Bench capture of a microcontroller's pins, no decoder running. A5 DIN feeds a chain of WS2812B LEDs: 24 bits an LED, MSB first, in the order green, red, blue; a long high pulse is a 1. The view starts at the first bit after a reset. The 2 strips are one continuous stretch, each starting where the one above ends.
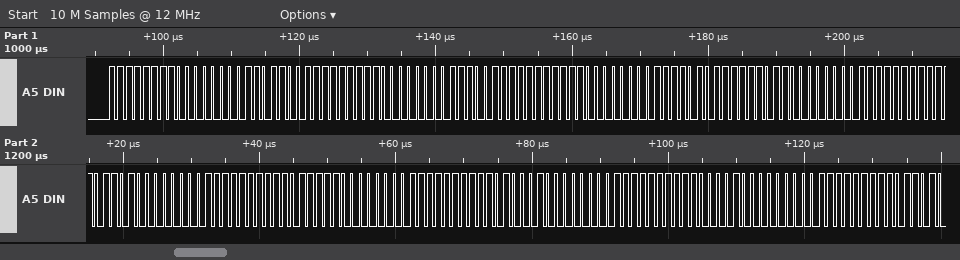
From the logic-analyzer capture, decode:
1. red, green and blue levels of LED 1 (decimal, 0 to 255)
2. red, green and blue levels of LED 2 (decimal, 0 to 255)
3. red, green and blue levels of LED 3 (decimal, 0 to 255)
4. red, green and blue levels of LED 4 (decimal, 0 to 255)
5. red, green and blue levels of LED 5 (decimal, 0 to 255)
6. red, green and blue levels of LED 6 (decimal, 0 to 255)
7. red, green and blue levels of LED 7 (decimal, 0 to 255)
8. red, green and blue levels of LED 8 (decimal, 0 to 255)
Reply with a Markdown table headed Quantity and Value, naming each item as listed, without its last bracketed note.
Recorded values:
| Quantity | Value |
|---|---|
| red, green and blue levels of LED 1 | 0, 255, 217 |
| red, green and blue levels of LED 2 | 0, 255, 231 |
| red, green and blue levels of LED 3 | 0, 255, 245 |
| red, green and blue levels of LED 4 | 0, 251, 255 |
| red, green and blue levels of LED 5 | 0, 237, 255 |
| red, green and blue levels of LED 6 | 0, 223, 255 |
| red, green and blue levels of LED 7 | 0, 209, 255 |
| red, green and blue levels of LED 8 | 0, 194, 255 |
